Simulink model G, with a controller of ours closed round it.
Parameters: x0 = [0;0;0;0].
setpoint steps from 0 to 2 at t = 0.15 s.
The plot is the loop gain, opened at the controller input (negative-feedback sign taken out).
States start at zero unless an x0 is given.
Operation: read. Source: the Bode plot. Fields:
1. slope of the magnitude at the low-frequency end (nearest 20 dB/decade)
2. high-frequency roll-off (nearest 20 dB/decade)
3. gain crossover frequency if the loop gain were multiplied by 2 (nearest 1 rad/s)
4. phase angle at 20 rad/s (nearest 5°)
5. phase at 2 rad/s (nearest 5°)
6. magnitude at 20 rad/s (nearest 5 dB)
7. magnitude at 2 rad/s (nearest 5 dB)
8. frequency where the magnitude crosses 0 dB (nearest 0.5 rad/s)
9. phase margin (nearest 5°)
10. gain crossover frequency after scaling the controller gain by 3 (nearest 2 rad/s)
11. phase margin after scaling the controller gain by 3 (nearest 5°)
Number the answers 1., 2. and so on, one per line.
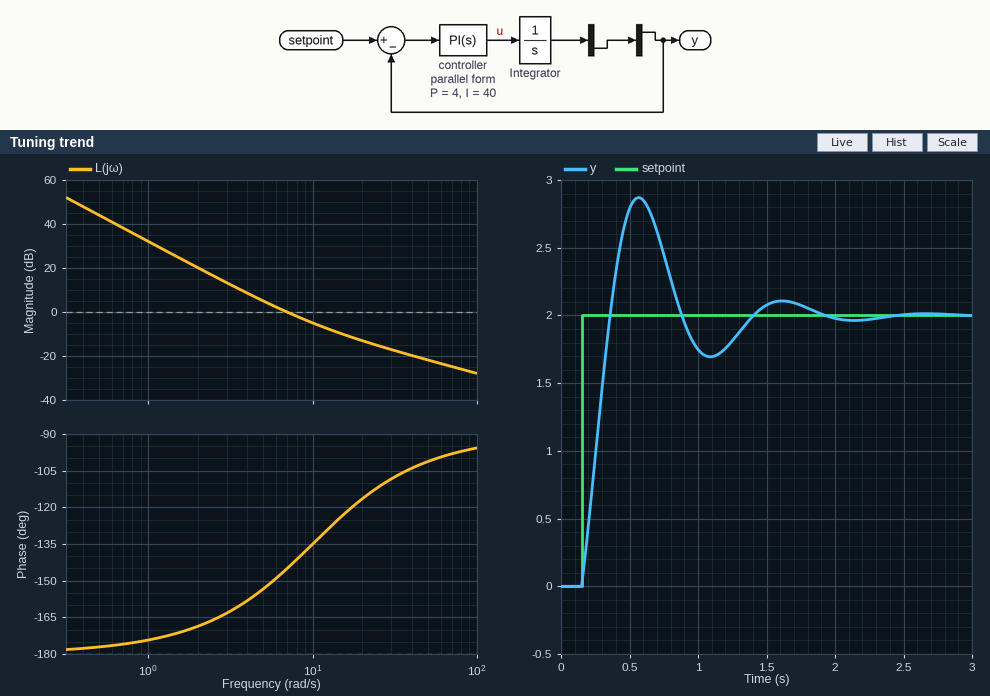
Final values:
1. -40 dB/decade
2. -20 dB/decade
3. 11 rad/s
4. -115°
5. -170°
6. -15 dB
7. 20 dB
8. 7.0 rad/s
9. 35°
10. 14 rad/s
11. 55°
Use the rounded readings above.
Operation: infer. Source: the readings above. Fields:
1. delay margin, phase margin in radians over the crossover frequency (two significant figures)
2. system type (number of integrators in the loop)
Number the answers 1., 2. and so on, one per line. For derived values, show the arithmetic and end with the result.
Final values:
1. 35 × π / 180 / 7 = 0.087 s
2. 2
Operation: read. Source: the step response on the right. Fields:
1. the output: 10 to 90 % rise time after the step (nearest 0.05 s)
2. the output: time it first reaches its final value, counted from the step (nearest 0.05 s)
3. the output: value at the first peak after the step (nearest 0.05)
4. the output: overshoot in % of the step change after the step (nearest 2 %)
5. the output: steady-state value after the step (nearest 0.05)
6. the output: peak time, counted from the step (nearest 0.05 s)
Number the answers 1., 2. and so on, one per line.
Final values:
1. 0.15 s
2. 0.20 s
3. 2.85
4. 44 %
5. 2.00
6. 0.40 s
